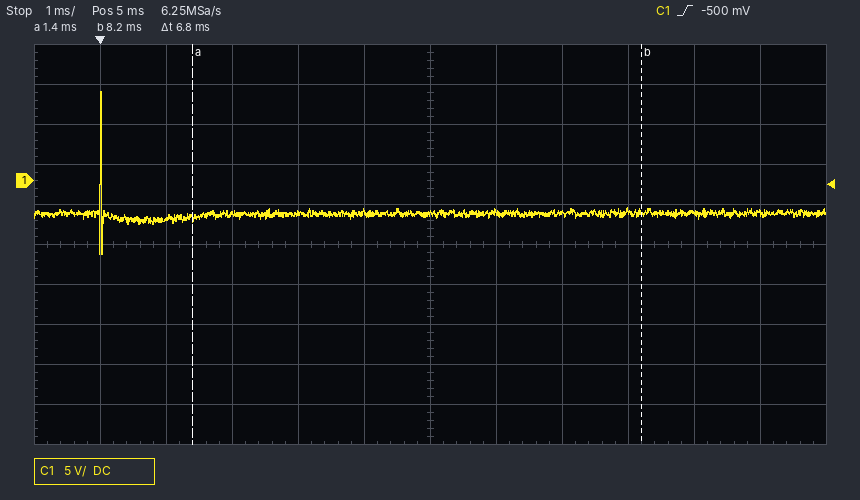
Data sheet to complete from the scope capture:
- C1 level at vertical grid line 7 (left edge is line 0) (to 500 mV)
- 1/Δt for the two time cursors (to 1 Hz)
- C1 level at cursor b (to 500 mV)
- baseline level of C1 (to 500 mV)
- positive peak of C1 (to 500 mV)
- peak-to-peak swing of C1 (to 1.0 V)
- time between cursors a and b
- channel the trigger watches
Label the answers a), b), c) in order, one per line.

a) -4.0 V
b) 147 Hz
c) -4.0 V
d) -4.0 V
e) 11.0 V
f) 20.0 V
g) 6.8 ms
h) C1
